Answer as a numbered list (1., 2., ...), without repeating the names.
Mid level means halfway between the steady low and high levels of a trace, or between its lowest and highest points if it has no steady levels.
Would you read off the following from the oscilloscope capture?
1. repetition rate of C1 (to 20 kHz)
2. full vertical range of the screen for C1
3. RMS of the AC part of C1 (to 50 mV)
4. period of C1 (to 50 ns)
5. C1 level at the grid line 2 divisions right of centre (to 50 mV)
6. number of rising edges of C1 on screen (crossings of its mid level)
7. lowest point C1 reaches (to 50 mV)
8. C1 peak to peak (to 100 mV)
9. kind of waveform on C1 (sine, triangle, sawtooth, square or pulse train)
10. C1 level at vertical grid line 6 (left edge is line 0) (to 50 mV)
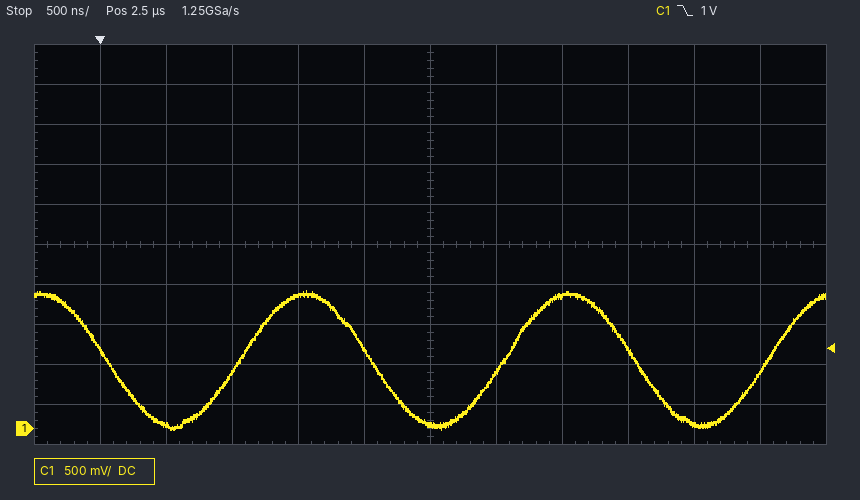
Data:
1. 500 kHz
2. 5 V
3. 600 mV
4. 2.00 µs
5. 1.65 V
6. 3
7. 0 mV
8. 1.70 V
9. sine
10. 50 mV
